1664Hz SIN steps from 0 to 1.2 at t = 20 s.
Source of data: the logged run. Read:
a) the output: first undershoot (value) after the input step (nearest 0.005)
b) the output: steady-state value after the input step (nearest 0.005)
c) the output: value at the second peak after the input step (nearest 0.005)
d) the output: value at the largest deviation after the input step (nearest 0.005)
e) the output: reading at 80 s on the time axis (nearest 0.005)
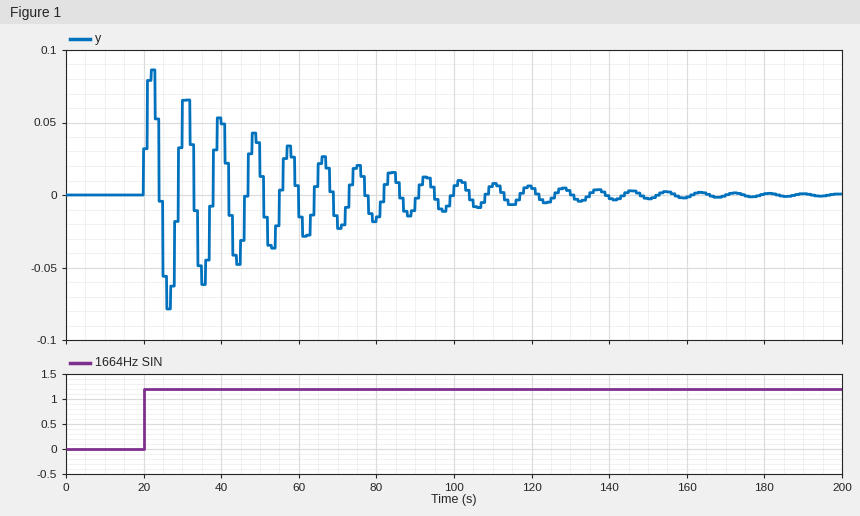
-0.080
0.000
0.065
0.085
-0.015
